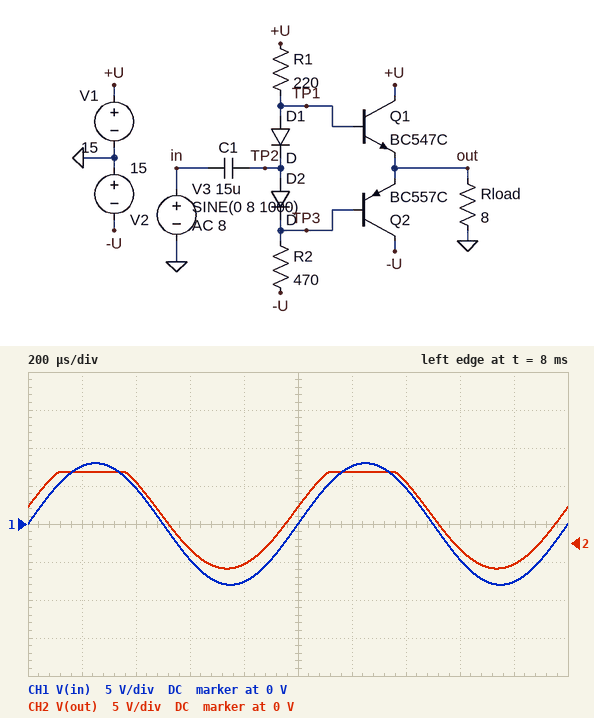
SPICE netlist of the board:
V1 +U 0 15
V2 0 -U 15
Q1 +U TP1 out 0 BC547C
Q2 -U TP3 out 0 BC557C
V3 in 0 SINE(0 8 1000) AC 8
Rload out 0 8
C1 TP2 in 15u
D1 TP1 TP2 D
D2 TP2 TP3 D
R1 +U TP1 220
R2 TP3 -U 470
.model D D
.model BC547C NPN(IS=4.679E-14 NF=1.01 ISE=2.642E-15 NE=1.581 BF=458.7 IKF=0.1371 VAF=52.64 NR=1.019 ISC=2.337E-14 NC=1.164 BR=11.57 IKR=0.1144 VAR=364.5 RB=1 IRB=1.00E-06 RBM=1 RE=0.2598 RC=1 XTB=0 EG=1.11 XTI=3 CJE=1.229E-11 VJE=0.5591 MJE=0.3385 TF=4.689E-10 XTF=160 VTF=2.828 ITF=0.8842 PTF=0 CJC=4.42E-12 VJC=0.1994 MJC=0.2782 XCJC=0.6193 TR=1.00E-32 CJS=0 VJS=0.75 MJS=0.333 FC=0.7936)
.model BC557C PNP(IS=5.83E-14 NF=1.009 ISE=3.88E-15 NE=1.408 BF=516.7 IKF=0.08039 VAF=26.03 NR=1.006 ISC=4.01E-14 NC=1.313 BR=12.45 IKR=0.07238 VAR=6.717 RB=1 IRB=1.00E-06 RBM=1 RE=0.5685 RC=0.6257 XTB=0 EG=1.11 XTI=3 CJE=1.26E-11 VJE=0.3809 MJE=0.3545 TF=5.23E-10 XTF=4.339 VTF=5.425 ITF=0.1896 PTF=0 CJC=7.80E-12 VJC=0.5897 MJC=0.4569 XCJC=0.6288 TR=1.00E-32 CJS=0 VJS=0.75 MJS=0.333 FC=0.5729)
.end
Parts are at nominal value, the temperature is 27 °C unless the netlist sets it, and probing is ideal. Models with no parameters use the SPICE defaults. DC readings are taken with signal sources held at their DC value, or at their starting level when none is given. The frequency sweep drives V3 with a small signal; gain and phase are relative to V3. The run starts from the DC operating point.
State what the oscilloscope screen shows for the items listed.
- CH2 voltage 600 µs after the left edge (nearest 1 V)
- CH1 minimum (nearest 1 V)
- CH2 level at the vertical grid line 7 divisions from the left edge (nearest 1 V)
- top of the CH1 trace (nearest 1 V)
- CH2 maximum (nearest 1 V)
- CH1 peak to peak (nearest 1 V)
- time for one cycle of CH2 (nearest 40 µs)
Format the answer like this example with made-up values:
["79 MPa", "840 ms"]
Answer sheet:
["-1 V", "-8 V", "8 V", "8 V", "9 V", "16 V", "1.00 ms"]
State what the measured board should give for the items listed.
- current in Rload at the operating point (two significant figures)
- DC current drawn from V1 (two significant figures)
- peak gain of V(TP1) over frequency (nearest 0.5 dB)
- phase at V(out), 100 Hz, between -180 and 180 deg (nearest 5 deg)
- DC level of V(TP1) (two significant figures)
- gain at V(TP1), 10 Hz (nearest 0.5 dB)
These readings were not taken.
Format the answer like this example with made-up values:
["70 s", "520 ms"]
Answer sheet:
["540 mA", "580 mA", "0 dB", "40 deg", "5.3 V", "-19.0 dB"]
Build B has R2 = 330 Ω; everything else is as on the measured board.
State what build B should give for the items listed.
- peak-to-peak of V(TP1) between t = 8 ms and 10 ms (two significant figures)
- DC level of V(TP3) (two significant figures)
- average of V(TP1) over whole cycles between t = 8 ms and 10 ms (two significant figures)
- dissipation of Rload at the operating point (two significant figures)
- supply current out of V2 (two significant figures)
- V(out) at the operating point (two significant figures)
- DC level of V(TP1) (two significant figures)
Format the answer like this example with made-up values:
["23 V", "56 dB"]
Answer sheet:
["15 V", "1.9 V", "3.0 V", "790 mW", "54 mA", "2.5 V", "3.4 V"]
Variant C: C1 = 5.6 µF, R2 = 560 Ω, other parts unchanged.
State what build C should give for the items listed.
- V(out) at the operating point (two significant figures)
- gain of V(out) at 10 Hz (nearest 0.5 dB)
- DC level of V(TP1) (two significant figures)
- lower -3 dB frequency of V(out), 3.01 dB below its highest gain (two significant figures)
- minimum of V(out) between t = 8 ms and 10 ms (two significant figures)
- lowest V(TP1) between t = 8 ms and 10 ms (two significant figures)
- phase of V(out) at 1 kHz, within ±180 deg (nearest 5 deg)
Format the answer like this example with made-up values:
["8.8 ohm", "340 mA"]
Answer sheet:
["5.0 V", "-28.0 dB", "6.0 V", "240 Hz", "-2.3 V", "-1.8 V", "15 deg"]
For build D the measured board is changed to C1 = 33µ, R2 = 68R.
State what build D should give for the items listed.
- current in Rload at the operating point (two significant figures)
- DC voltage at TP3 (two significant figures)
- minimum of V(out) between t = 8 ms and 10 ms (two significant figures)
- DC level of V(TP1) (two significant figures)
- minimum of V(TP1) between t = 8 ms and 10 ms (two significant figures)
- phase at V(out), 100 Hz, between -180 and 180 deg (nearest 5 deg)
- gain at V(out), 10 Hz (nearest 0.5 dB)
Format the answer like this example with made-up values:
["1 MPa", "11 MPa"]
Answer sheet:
["790 mA", "-7.6 V", "-10 V", "-6.1 V", "-14 V", "50 deg", "-22.0 dB"]
